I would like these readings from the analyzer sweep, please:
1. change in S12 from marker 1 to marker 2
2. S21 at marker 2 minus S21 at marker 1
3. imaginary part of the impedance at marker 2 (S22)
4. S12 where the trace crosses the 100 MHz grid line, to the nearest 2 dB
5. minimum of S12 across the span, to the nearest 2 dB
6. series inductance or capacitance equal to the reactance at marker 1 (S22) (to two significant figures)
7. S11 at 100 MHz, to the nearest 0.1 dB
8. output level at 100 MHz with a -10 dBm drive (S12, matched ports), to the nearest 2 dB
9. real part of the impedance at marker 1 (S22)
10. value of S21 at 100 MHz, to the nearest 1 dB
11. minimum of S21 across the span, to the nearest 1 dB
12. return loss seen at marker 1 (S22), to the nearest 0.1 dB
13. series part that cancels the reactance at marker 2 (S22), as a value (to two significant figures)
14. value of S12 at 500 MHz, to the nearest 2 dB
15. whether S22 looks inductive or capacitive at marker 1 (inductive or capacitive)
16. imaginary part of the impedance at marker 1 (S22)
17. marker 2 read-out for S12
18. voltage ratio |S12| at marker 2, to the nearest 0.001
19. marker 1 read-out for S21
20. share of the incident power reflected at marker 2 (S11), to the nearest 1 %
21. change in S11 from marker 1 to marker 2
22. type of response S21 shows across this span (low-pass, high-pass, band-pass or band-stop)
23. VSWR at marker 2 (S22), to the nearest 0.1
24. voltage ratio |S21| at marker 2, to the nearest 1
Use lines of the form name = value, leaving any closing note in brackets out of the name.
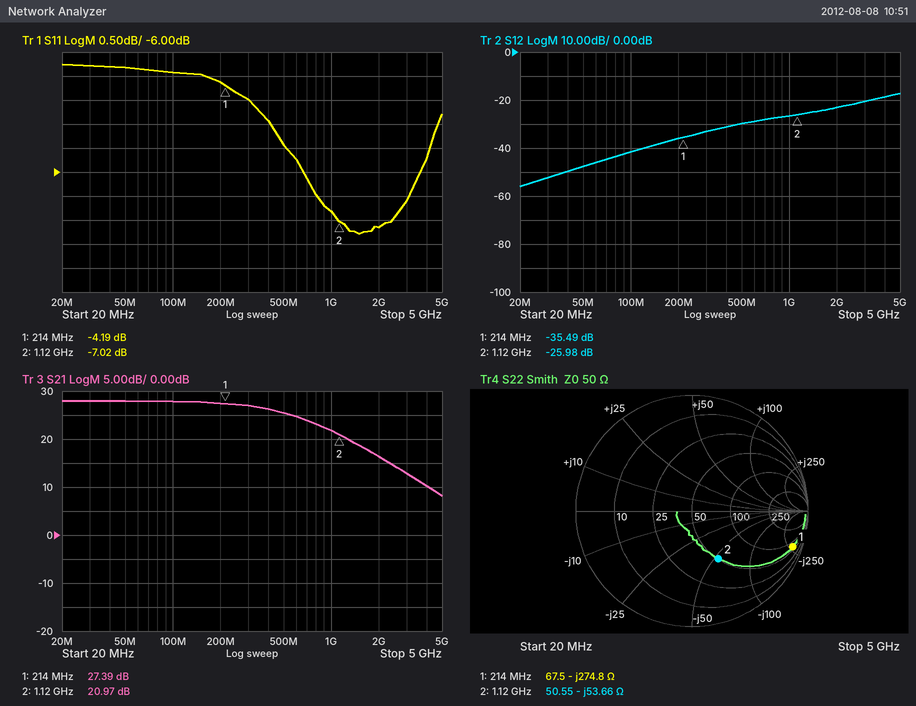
change in S12 from marker 1 to marker 2 = 9.51 dB
S21 at marker 2 minus S21 at marker 1 = -6.42 dB
imaginary part of the impedance at marker 2 = -53.66 Ω
S12 where the trace crosses the 100 MHz grid line, to the nearest 2 dB = -42 dB
minimum of S12 across the span, to the nearest 2 dB = -56 dB
series inductance or capacitance equal to the reactance at marker 1 (S22) = 2.7 pF
S11 at 100 MHz, to the nearest 0.1 dB = -3.9 dB
output level at 100 MHz with a -10 dBm drive (S12, matched ports), to the nearest 2 dB = -52 dBm
real part of the impedance at marker 1 = 67.5 Ω
value of S21 at 100 MHz, to the nearest 1 dB = 28 dB
minimum of S21 across the span, to the nearest 1 dB = 8 dB
return loss seen at marker 1 (S22), to the nearest 0.1 dB = 0.7 dB
series part that cancels the reactance at marker 2 (S22), as a value = 7.6 nH
value of S12 at 500 MHz, to the nearest 2 dB = -30 dB
whether S22 looks inductive or capacitive at marker 1 = capacitive
imaginary part of the impedance at marker 1 = -274.8 Ω
marker 2 read-out for S12 = -25.98 dB
voltage ratio |S12| at marker 2, to the nearest 0.001 = 0.050
marker 1 read-out for S21 = 27.39 dB
share of the incident power reflected at marker 2 (S11), to the nearest 1 % = 20 %
change in S11 from marker 1 to marker 2 = -2.83 dB
type of response S21 shows across this span = low-pass
VSWR at marker 2 (S22), to the nearest 0.1 = 2.8
voltage ratio |S21| at marker 2, to the nearest 1 = 11
